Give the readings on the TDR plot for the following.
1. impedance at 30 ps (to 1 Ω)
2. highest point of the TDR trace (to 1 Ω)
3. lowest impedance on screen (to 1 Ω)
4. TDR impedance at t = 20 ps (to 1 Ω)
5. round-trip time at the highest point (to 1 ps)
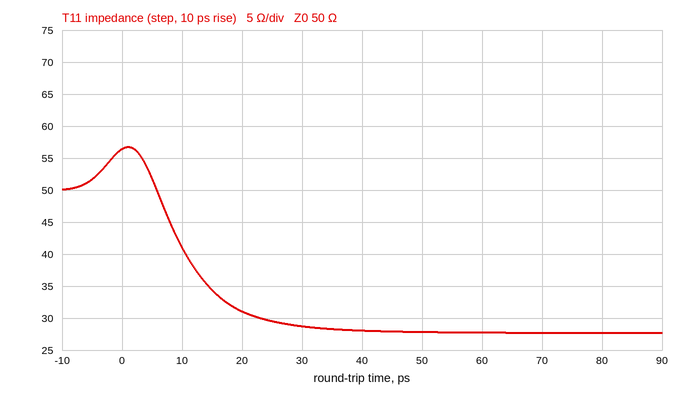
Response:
29 Ω
57 Ω
28 Ω
31 Ω
1 ps
